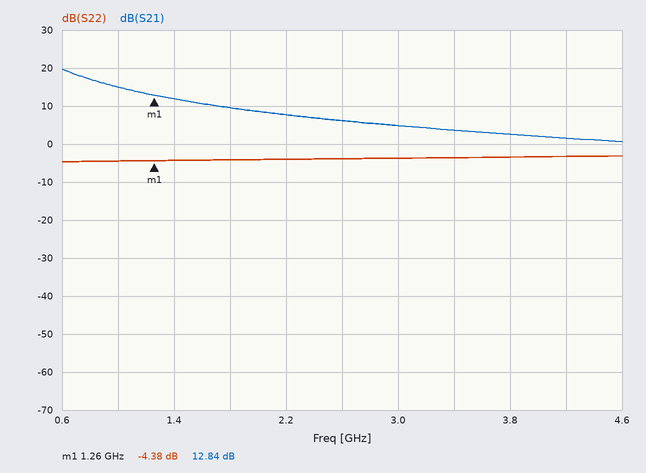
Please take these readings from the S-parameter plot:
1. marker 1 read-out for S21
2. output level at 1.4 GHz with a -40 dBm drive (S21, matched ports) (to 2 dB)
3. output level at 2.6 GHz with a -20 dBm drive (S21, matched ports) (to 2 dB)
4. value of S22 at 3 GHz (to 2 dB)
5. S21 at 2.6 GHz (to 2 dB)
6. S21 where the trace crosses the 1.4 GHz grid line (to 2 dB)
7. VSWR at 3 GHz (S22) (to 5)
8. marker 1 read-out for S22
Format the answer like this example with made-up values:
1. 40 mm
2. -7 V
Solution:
1. 12.84 dB
2. -28 dBm
3. -14 dBm
4. -4 dB
5. 6 dB
6. 12 dB
7. 5
8. -4.38 dB
